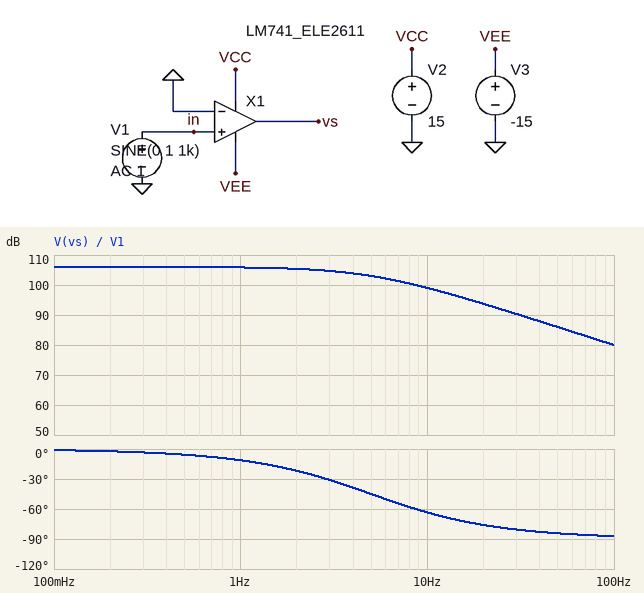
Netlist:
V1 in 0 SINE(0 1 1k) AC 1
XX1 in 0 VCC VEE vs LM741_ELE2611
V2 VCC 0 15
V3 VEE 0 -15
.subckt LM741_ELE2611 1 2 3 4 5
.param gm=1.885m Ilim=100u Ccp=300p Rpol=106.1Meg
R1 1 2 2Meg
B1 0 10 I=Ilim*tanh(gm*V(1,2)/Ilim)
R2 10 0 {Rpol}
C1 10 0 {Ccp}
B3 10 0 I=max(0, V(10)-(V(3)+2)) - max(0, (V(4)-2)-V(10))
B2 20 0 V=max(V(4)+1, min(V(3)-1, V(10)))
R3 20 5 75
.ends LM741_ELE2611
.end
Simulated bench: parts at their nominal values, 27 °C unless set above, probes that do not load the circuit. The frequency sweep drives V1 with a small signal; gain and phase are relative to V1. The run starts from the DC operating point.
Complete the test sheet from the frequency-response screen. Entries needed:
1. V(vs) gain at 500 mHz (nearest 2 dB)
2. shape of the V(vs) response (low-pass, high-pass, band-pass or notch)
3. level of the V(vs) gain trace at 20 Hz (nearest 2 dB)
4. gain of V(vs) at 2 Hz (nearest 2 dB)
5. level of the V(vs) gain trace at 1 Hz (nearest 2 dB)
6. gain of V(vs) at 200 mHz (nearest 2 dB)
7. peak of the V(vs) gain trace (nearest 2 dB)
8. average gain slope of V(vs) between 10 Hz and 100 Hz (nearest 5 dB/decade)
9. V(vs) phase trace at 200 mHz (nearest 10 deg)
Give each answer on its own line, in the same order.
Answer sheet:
106 dB
low-pass
94 dB
106 dB
106 dB
106 dB
106 dB
-20 dB/decade
0 deg
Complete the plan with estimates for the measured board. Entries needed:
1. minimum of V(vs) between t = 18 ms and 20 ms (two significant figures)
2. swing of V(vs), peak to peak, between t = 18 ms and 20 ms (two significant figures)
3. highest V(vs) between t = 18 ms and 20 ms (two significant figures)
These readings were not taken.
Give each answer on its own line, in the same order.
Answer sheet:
-14 V
28 V
14 V
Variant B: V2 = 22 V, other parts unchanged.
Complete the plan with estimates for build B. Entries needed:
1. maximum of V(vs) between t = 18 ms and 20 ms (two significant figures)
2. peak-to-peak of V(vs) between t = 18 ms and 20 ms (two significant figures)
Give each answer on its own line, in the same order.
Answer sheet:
21 V
35 V
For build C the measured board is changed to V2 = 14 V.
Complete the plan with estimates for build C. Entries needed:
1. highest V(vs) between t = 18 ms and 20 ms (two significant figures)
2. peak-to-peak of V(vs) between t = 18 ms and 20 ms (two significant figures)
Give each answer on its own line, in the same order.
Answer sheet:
13 V
27 V
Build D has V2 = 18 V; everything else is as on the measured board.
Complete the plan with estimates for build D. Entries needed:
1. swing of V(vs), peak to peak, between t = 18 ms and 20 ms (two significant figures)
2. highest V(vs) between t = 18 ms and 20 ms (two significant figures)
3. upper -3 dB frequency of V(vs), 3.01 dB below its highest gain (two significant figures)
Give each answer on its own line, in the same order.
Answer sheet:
31 V
17 V
5.0 Hz
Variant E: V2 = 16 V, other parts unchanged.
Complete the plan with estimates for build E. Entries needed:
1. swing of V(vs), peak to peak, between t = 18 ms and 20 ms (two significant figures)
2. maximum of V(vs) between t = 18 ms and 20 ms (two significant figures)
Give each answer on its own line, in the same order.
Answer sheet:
29 V
15 V
